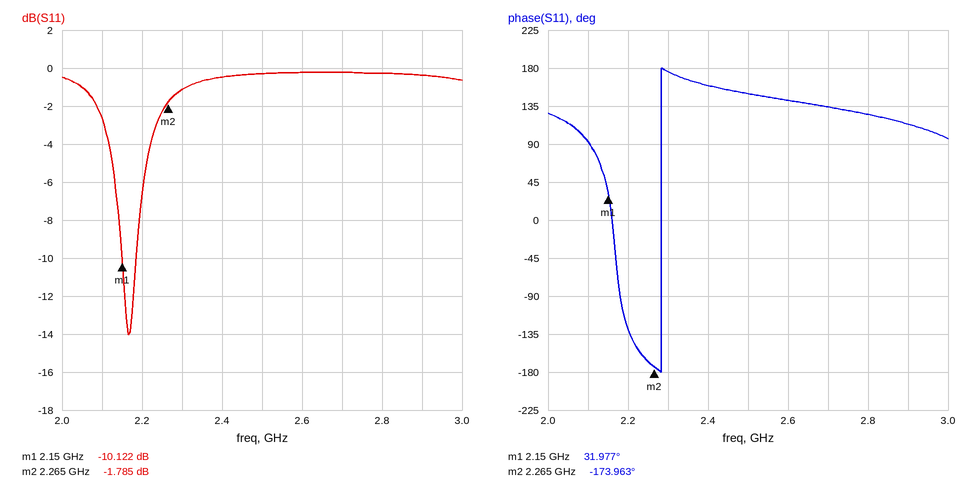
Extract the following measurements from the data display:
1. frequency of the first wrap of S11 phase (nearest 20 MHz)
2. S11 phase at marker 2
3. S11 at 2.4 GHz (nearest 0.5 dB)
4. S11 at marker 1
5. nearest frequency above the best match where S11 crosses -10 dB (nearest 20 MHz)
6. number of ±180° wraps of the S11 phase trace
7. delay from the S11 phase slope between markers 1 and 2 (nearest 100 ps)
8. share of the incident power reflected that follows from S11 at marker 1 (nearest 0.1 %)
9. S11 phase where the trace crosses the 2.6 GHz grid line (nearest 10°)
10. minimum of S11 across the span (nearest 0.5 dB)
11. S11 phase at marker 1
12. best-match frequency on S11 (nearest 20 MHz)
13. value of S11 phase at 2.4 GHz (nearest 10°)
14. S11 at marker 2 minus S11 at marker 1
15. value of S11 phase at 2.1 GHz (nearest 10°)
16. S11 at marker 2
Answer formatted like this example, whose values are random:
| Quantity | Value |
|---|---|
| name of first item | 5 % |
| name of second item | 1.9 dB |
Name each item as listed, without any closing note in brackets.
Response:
| Quantity | Value |
|---|---|
| frequency of the first wrap of S11 phase | 2.28 GHz |
| S11 phase at marker 2 | -173.963° |
| S11 at 2.4 GHz | -0.5 dB |
| S11 at marker 1 | -10.122 dB |
| nearest frequency above the best match where S11 crosses -10 dB | 2.18 GHz |
| number of ±180° wraps of the S11 phase trace | 1 |
| delay from the S11 phase slope between markers 1 and 2 | 5.0 ns |
| share of the incident power reflected that follows from S11 at marker 1 | 9.7 % |
| S11 phase where the trace crosses the 2.6 GHz grid line | 140° |
| minimum of S11 across the span | -14.0 dB |
| S11 phase at marker 1 | 31.977° |
| best-match frequency on S11 | 2.16 GHz |
| value of S11 phase at 2.4 GHz | 160° |
| S11 at marker 2 minus S11 at marker 1 | 8.337 dB |
| value of S11 phase at 2.1 GHz | 90° |
| S11 at marker 2 | -1.785 dB |
